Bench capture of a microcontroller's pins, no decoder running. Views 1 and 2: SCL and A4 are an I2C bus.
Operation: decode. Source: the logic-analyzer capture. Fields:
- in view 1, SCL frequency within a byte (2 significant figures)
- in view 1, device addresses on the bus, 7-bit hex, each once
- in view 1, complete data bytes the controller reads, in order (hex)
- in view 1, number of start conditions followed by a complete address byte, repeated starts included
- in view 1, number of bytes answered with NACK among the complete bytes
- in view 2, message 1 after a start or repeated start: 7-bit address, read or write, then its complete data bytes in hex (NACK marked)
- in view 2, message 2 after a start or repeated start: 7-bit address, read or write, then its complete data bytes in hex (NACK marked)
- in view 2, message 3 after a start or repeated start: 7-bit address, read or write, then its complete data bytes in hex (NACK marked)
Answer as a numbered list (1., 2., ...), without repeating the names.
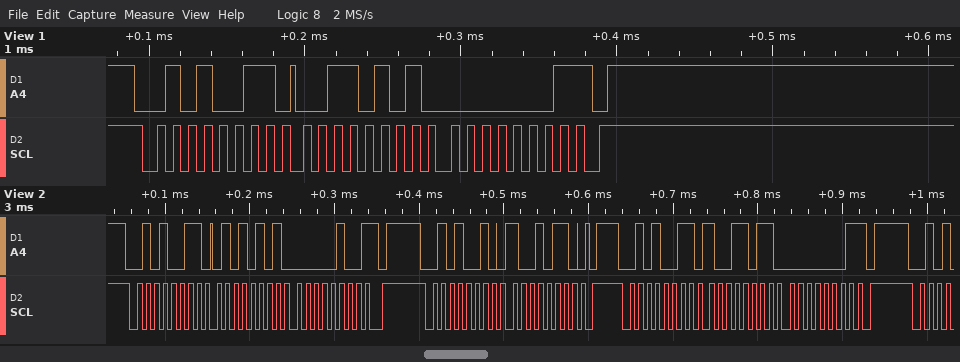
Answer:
1. 100 kHz
2. 0x29
3. 35 01
4. 1
5. 1
6. 0x29 read: 55 04 NACK
7. 0x29 write: 96
8. 0x29 read: 9B 01 NACK
